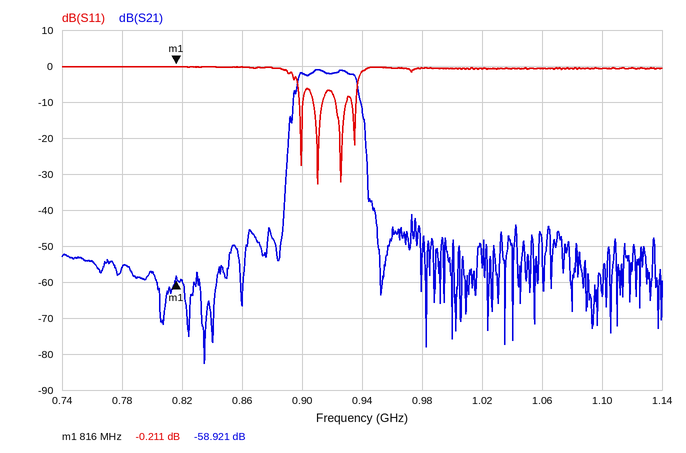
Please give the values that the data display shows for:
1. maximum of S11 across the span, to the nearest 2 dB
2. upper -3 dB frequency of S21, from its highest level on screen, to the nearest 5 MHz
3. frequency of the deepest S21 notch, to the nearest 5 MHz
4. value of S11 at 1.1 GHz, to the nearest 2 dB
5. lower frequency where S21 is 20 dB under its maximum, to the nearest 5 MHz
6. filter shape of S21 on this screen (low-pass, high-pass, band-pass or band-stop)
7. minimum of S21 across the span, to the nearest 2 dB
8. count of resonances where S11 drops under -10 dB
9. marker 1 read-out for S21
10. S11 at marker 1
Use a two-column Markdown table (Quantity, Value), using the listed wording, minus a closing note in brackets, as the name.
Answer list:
| Quantity | Value |
|---|---|
| maximum of S11 across the span, to the nearest 2 dB | 0 dB |
| upper -3 dB frequency of S21, from its highest level on screen, to the nearest 5 MHz | 935 MHz |
| frequency of the deepest S21 notch, to the nearest 5 MHz | 835 MHz |
| value of S11 at 1.1 GHz, to the nearest 2 dB | 0 dB |
| lower frequency where S21 is 20 dB under its maximum, to the nearest 5 MHz | 890 MHz |
| filter shape of S21 on this screen | band-pass |
| minimum of S21 across the span, to the nearest 2 dB | -82 dB |
| count of resonances where S11 drops under -10 dB | 4 |
| marker 1 read-out for S21 | -58.921 dB |
| S11 at marker 1 | -0.211 dB |
